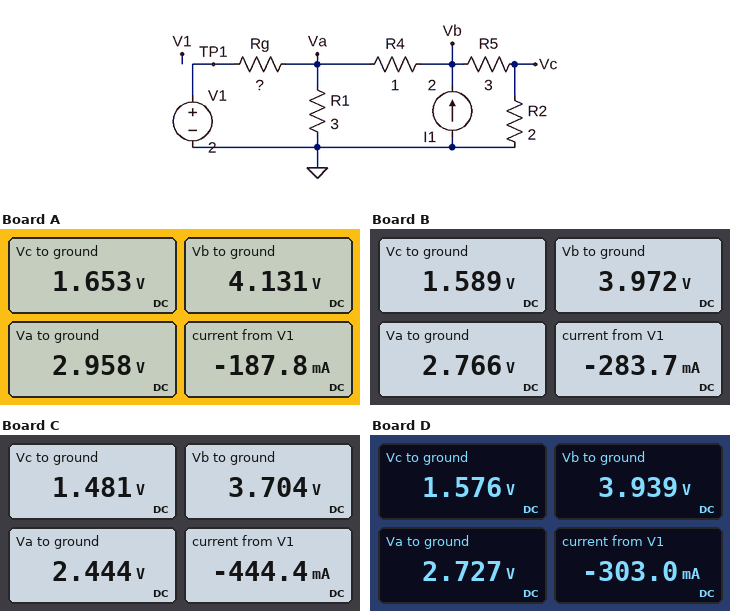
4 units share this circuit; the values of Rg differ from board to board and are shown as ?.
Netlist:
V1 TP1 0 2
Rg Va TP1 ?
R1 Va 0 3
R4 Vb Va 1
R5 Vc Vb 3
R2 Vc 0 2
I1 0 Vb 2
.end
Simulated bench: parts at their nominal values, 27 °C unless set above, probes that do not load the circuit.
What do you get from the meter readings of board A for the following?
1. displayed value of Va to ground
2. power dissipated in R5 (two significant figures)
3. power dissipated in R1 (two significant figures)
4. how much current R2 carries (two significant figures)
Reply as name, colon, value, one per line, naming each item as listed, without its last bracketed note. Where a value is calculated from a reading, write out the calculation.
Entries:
displayed value of Va to ground: 2.958 V
power dissipated in R5: (4.131 V - 1.653 V)^2 / 3 Ω = 2.0 W
power dissipated in R1: (2.958 V)^2 / 3 Ω = 2.9 W
how much current R2 carries: (1.653 V) / 2 Ω = 830 mA
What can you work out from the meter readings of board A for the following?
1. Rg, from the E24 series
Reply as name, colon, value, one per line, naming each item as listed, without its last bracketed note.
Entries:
Rg, from the E24 series: 5.1 Ω
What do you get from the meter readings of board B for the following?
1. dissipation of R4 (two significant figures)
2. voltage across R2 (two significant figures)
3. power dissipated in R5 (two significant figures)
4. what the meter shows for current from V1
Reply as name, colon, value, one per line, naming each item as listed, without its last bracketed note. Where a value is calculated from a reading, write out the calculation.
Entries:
dissipation of R4: (3.972 V - 2.766 V)^2 / 1 Ω = 1.5 W
voltage across R2: 1.589 V = 1.6 V
power dissipated in R5: (3.972 V - 1.589 V)^2 / 3 Ω = 1.9 W
what the meter shows for current from V1: -283.7 mA
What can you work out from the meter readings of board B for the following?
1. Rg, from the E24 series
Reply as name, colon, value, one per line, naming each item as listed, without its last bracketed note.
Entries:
Rg, from the E24 series: 2.7 Ω
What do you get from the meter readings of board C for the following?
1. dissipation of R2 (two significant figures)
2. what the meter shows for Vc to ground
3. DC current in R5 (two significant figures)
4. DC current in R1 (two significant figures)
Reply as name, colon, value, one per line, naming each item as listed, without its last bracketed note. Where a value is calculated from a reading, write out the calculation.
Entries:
dissipation of R2: (1.481 V)^2 / 2 Ω = 1.1 W
what the meter shows for Vc to ground: 1.481 V
DC current in R5: (3.704 V - 1.481 V) / 3 Ω = 740 mA
DC current in R1: (2.444 V) / 3 Ω = 810 mA
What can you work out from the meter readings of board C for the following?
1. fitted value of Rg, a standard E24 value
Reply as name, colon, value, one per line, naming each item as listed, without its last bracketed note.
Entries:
fitted value of Rg, a standard E24 value: 1 Ω
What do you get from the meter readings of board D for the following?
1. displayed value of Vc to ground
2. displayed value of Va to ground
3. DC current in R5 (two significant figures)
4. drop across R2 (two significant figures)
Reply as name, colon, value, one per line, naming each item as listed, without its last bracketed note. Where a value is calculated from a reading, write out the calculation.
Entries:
displayed value of Vc to ground: 1.576 V
displayed value of Va to ground: 2.727 V
DC current in R5: (3.939 V - 1.576 V) / 3 Ω = 790 mA
drop across R2: 1.576 V = 1.6 V
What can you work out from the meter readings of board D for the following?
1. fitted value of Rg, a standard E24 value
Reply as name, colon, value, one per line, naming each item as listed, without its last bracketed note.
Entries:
fitted value of Rg, a standard E24 value: 2.4 Ω
